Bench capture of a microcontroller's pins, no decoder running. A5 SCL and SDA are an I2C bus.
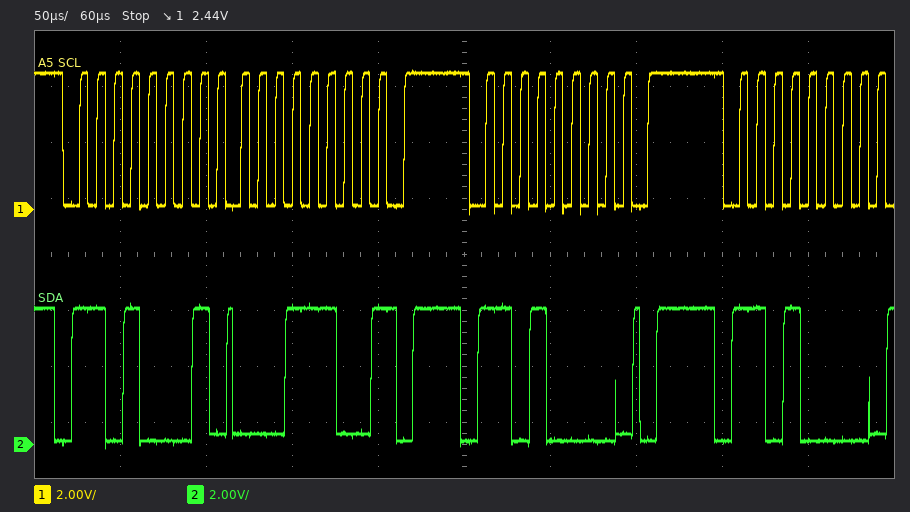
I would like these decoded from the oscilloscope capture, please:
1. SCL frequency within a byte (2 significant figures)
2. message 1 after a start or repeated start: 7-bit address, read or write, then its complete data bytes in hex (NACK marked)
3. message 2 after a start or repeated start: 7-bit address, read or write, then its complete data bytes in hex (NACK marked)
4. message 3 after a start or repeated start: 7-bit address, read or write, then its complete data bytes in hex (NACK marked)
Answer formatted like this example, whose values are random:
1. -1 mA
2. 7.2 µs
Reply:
1. 100 kHz
2. 0x68 read: 1C NACK
3. 0x68 write
4. 0x68 write
